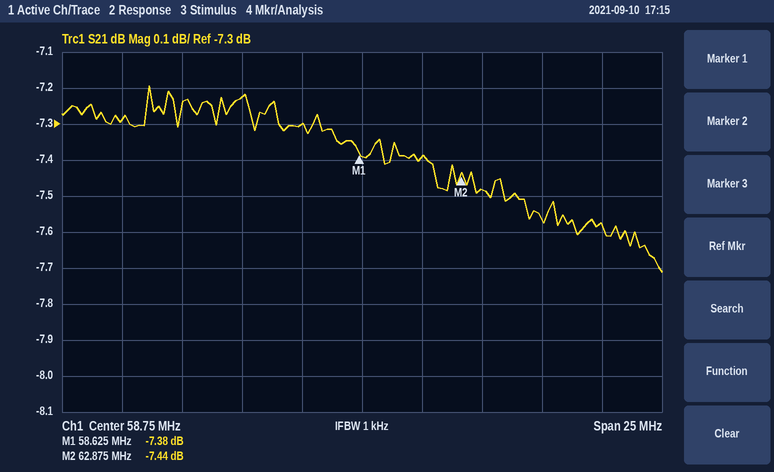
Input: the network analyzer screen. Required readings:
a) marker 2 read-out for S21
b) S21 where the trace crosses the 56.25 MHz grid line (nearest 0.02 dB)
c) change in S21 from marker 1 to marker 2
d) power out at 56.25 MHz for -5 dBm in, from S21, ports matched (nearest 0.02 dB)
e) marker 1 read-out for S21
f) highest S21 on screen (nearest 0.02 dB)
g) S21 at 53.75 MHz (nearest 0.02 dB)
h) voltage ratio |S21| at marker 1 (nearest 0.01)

-7.44 dB
-7.30 dB
-0.06 dB
-12.30 dBm
-7.38 dB
-7.20 dB
-7.22 dB
0.43
